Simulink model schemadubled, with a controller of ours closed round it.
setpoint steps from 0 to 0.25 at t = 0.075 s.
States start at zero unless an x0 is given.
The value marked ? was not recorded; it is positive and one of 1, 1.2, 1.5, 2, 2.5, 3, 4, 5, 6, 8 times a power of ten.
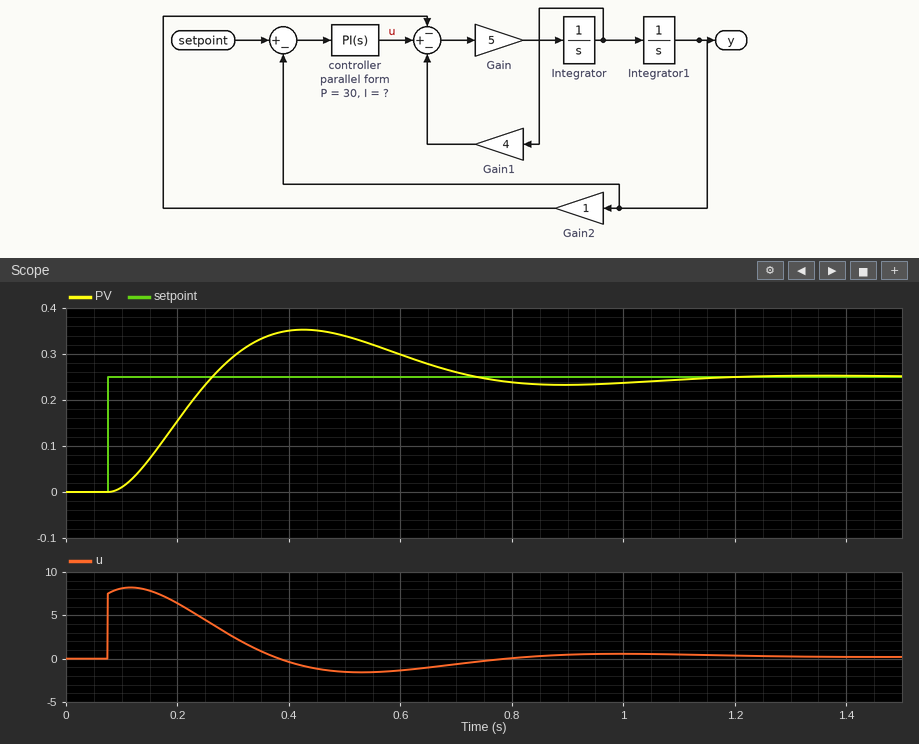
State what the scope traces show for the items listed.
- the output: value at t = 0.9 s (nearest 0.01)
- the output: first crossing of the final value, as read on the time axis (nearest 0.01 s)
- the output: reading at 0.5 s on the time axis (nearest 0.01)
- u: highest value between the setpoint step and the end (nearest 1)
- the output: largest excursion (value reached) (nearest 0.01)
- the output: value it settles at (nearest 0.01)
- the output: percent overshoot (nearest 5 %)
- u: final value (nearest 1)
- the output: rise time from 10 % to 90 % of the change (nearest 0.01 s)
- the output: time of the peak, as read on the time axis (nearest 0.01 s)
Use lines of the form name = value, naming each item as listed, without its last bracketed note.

the output: value at t = 0.9 s = 0.23
the output: first crossing of the final value, as read on the time axis = 0.26 s
the output: reading at 0.5 s on the time axis = 0.34
u: highest value between the setpoint step and the end = 8
the output: largest excursion (value reached) = 0.35
the output: value it settles at = 0.25
the output: percent overshoot = 40 %
u: final value = 0
the output: rise time from 10 % to 90 % of the change = 0.13 s
the output: time of the peak, as read on the time axis = 0.43 s
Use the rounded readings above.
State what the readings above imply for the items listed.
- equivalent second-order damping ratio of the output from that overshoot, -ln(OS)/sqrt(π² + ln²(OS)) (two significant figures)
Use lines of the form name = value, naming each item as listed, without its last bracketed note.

equivalent second-order damping ratio of the output from that overshoot, -ln(OS)/sqrt(π² + ln²(OS)) = 0.28
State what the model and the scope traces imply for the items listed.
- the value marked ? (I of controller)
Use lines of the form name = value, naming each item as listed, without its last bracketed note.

the value marked ? = 150
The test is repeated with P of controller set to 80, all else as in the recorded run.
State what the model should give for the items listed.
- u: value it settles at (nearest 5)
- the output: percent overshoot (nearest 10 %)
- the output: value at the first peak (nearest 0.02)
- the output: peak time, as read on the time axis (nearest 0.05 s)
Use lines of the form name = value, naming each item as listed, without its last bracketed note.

u: value it settles at = 0
the output: percent overshoot = 30 %
the output: value at the first peak = 0.32
the output: peak time, as read on the time axis = 0.25 s
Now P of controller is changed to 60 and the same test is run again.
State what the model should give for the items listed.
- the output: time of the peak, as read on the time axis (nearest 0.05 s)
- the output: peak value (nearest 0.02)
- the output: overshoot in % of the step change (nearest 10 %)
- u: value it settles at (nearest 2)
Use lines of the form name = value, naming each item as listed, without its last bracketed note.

the output: time of the peak, as read on the time axis = 0.30 s
the output: peak value = 0.32
the output: overshoot in % of the step change = 30 %
u: value it settles at = 0
